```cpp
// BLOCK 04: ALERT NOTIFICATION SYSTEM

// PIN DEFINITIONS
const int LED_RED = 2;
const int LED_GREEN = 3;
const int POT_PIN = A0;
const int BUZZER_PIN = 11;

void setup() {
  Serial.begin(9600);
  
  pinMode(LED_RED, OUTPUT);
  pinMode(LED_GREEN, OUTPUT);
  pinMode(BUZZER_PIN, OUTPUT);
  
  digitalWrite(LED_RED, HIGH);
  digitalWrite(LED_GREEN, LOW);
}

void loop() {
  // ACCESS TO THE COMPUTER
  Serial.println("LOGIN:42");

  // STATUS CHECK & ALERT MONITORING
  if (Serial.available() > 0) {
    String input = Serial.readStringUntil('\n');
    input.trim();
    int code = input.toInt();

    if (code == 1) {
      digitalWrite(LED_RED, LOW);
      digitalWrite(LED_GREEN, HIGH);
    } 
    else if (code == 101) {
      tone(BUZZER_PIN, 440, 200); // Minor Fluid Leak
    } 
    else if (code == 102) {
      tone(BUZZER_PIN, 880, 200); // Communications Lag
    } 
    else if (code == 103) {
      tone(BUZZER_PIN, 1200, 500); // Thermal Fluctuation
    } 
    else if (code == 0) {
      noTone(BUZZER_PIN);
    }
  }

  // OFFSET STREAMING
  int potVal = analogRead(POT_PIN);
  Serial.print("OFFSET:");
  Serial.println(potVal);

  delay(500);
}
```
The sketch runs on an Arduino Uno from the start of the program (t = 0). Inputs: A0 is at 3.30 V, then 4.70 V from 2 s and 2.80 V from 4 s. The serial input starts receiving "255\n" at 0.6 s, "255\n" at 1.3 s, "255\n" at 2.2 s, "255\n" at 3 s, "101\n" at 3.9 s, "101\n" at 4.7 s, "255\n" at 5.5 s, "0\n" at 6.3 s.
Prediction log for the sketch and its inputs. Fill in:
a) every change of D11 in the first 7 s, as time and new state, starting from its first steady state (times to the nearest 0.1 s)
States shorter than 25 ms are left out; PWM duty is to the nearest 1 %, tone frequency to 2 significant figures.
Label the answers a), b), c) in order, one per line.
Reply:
a) 0 s low; 4 s tone 440 Hz; 4.2 s low; 5 s tone 440 Hz; 5.2 s low
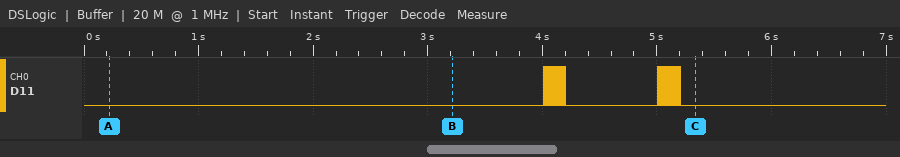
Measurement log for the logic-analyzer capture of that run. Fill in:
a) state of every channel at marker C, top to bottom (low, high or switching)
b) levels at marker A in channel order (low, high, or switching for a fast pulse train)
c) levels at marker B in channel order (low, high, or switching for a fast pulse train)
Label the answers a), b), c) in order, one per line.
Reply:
a) D11 low
b) D11 low
c) D11 low
